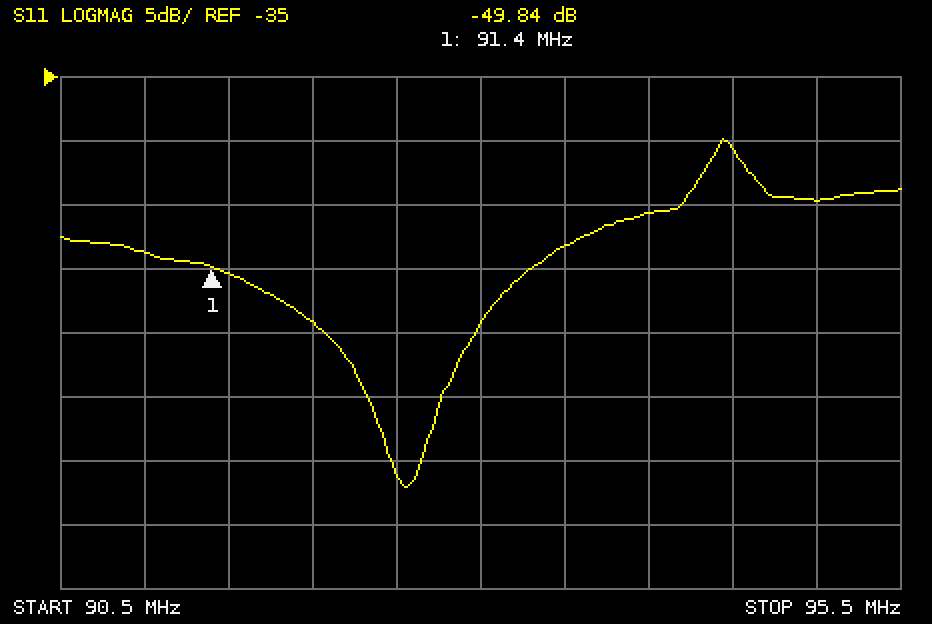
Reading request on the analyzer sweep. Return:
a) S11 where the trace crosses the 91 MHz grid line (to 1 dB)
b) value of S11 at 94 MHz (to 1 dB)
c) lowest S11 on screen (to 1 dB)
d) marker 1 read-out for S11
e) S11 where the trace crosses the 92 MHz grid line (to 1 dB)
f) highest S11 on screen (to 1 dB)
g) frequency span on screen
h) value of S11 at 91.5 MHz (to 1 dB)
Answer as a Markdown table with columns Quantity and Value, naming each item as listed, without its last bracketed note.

| Quantity | Value |
|---|---|
| S11 where the trace crosses the 91 MHz grid line | -49 dB |
| value of S11 at 94 MHz | -46 dB |
| lowest S11 on screen | -67 dB |
| marker 1 read-out for S11 | -49.84 dB |
| S11 where the trace crosses the 92 MHz grid line | -54 dB |
| highest S11 on screen | -40 dB |
| frequency span on screen | 5 MHz |
| value of S11 at 91.5 MHz | -50 dB |
